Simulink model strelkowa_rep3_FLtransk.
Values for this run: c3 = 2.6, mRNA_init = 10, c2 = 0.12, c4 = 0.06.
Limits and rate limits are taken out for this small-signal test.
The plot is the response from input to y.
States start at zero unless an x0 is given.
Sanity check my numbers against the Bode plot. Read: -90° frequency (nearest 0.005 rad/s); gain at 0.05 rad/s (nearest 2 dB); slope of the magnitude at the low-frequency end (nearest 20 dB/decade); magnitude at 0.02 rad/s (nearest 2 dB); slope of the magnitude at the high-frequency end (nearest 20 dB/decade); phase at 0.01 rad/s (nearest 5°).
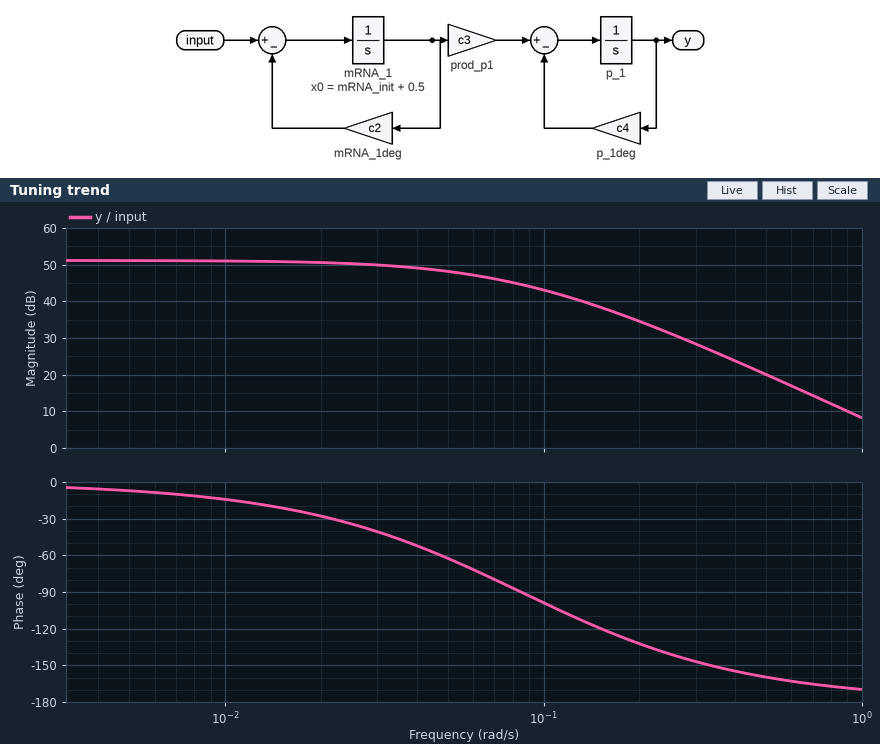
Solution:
0.085 rad/s
48 dB
0 dB/decade
50 dB
-40 dB/decade
-15°
